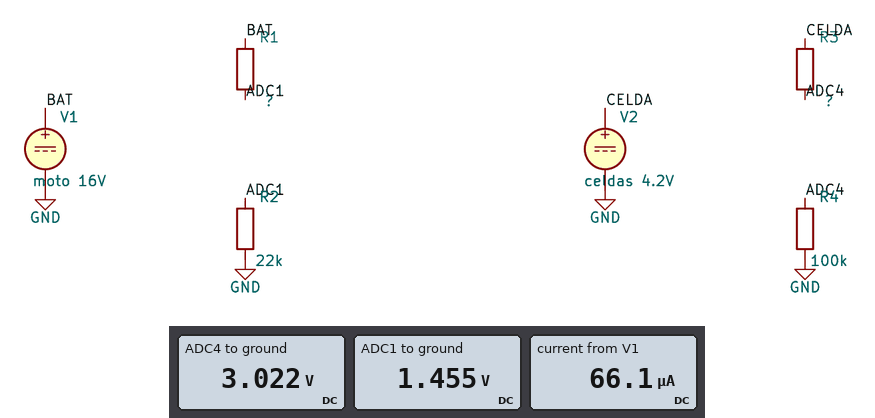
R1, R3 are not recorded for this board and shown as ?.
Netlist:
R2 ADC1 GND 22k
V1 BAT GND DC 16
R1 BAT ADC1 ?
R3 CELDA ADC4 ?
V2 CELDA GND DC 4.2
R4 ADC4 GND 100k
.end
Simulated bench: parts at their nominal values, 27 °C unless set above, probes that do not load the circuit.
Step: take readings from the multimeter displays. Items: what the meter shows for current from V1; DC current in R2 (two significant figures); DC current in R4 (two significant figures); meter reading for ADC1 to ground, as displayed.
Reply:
66.1 µA
66 µA
30 µA
1.455 V
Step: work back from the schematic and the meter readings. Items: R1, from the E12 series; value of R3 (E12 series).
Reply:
220 kΩ
39 kΩ
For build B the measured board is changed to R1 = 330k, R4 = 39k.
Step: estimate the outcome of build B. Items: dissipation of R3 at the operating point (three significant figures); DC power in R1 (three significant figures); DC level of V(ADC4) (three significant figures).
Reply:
113 µW
682 µW
2.10 V
